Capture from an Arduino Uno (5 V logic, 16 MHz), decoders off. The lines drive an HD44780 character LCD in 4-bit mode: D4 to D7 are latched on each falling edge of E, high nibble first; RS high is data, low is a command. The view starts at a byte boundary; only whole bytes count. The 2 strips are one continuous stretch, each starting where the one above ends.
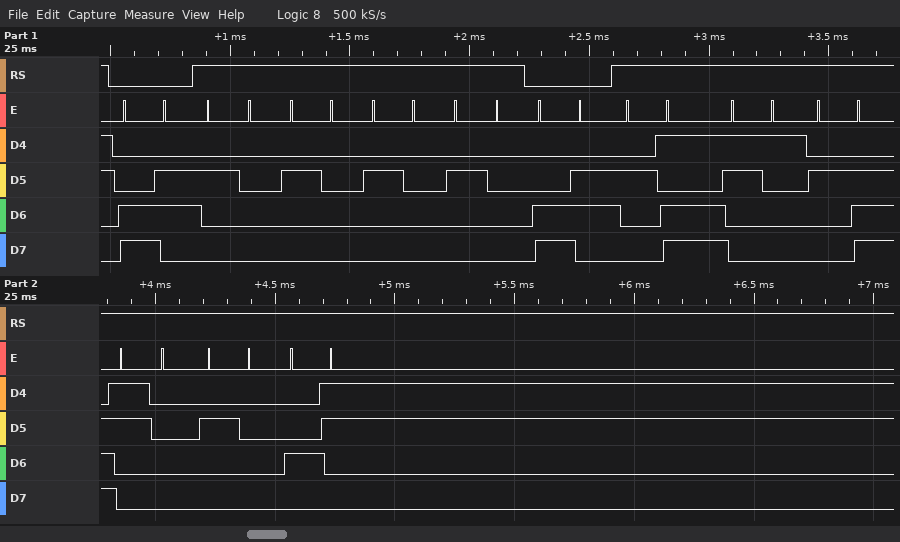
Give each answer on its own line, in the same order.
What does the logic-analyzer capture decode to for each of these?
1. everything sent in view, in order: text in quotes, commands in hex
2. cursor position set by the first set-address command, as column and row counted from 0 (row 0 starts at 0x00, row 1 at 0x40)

0xC6 "    " 0xC6 "-1.0 C"
column 6, row 1
